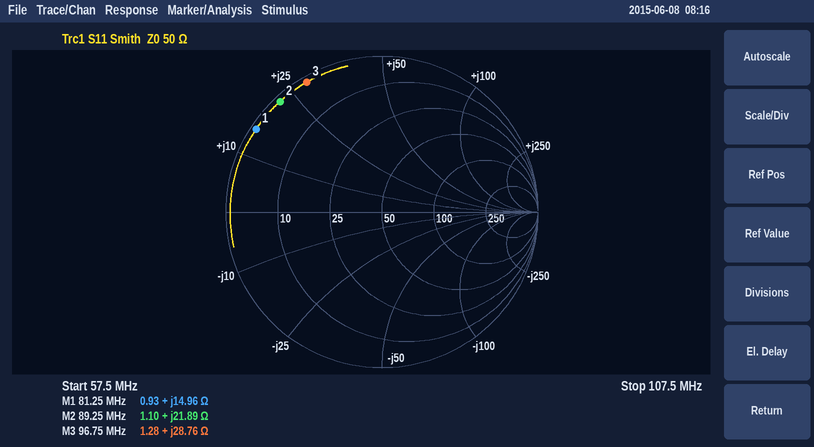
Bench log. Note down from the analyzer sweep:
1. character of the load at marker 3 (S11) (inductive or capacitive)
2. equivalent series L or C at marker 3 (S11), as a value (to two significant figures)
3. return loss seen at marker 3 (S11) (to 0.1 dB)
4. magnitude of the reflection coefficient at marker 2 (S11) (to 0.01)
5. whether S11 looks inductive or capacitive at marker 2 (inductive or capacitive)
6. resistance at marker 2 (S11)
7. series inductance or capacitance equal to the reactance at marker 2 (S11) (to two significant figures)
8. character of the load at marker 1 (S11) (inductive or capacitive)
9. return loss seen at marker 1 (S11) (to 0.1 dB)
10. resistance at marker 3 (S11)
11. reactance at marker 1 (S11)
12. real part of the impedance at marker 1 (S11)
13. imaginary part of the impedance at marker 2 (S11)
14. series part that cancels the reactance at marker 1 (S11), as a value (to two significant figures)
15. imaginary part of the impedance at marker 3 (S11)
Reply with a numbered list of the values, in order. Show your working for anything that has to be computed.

1. inductive
2. L = 28.76 Ω/(2π × 96.75 MHz) ≈ 47 nH
3. 0.3 dB
4. 0.96
5. inductive
6. 1.10 Ω
7. L = 21.89 Ω/(2π × 89.25 MHz) ≈ 39 nH
8. inductive
9. 0.3 dB
10. 1.28 Ω
11. +14.96 Ω
12. 0.93 Ω
13. +21.89 Ω
14. C = 1/(2π × 81.25 MHz × 14.96 Ω) ≈ 131 pF, so 130 pF to two significant figures
15. +28.76 Ω
